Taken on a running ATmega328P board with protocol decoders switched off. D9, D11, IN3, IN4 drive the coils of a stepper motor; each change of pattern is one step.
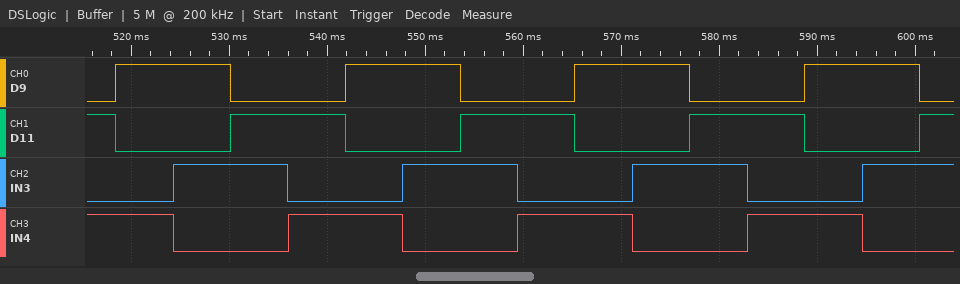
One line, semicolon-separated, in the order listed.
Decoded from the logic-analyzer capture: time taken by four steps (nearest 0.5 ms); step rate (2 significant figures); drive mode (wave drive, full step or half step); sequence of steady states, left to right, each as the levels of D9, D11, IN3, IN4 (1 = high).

23.5 ms; 170 steps/s; full step; 0101 1001 1010 0110 0101 1001 1010 0110 0101 1001 1010 0110 0101 1001 1010 0110
